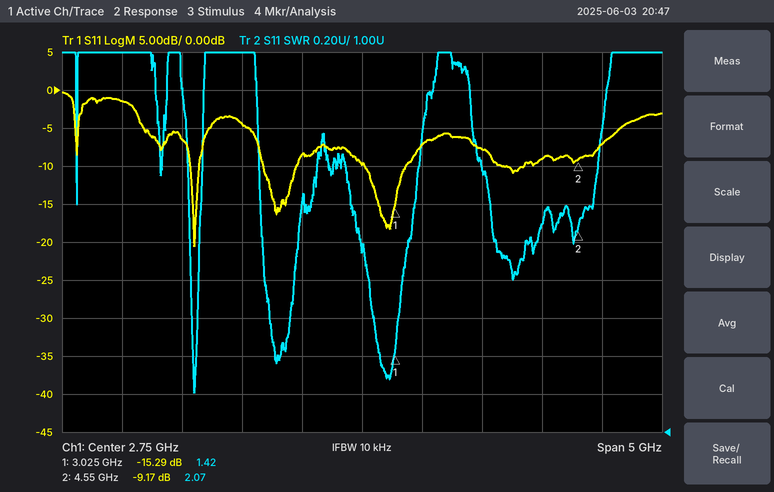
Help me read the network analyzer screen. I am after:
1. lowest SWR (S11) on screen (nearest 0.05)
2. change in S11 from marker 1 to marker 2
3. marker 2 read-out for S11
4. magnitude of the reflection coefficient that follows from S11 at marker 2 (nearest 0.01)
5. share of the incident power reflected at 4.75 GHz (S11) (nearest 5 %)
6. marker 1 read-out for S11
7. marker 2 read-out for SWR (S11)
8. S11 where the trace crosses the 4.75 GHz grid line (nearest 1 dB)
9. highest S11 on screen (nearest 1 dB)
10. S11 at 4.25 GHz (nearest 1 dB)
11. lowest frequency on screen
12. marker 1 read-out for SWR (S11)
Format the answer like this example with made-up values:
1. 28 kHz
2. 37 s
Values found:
1. 1.20
2. 6.12 dB
3. -9.17 dB
4. 0.35
5. 20 %
6. -15.29 dB
7. 2.07
8. -7 dB
9. 0 dB
10. -9 dB
11. 250 MHz
12. 1.42
